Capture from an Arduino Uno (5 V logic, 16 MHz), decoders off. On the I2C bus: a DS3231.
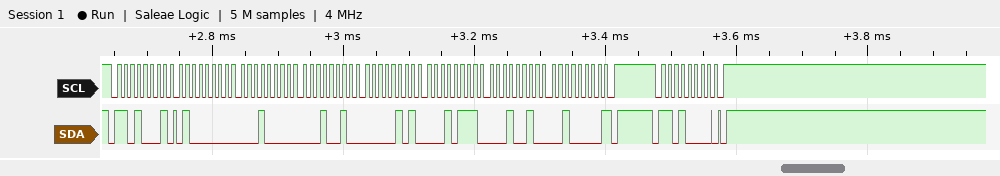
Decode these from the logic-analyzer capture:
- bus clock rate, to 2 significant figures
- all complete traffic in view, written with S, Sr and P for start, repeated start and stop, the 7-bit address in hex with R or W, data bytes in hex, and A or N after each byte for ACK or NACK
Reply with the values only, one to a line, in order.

100 kHz
S 68R A 40 A 10 A 12 A 05 A 17 A 12 A 20 N P S 68W A P
